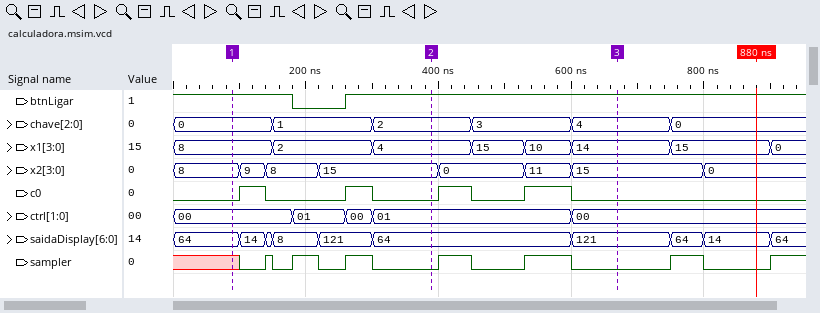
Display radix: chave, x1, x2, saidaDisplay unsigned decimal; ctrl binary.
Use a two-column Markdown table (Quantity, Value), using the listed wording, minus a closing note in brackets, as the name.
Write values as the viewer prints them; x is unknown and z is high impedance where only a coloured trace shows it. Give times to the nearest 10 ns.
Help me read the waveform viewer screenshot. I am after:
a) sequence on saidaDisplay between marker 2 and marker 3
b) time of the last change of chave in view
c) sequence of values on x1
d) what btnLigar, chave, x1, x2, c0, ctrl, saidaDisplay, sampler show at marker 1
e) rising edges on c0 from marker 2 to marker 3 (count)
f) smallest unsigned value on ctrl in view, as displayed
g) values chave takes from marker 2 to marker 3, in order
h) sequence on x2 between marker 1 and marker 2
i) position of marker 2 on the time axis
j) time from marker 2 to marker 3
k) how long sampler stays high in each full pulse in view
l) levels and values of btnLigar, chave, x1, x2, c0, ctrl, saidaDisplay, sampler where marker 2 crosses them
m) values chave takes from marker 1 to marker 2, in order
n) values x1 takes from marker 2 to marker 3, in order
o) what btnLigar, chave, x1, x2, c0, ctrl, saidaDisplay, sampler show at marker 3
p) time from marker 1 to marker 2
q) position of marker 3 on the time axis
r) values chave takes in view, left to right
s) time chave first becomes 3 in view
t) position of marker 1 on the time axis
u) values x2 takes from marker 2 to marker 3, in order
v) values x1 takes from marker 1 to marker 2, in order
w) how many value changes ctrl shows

| Quantity | Value |
|---|---|
| sequence on saidaDisplay between marker 2 and marker 3 | 64, 121 |
| time of the last change of chave in view | 750 ns |
| sequence of values on x1 | 8, 2, 4, 15, 10, 14, 15, 0 |
| what btnLigar, chave, x1, x2, c0, ctrl, saidaDisplay, sampler show at marker 1 | btnLigar=1, chave=0, x1=8, x2=8, c0=0, ctrl=00, saidaDisplay=64, sampler=x |
| rising edges on c0 from marker 2 to marker 3 | 2 |
| smallest unsigned value on ctrl in view, as displayed | 00 |
| values chave takes from marker 2 to marker 3, in order | 2, 3, 4 |
| sequence on x2 between marker 1 and marker 2 | 8, 9, 8, 15 |
| position of marker 2 on the time axis | 390 ns |
| time from marker 2 to marker 3 | 280 ns |
| how long sampler stays high in each full pulse in view | 10 ns, 40 ns, 40 ns, 50 ns, 70 ns, 50 ns |
| levels and values of btnLigar, chave, x1, x2, c0, ctrl, saidaDisplay, sampler where marker 2 crosses them | btnLigar=1, chave=2, x1=4, x2=15, c0=0, ctrl=01, saidaDisplay=64, sampler=0 |
| values chave takes from marker 1 to marker 2, in order | 0, 1, 2 |
| values x1 takes from marker 2 to marker 3, in order | 4, 15, 10, 14 |
| what btnLigar, chave, x1, x2, c0, ctrl, saidaDisplay, sampler show at marker 3 | btnLigar=1, chave=4, x1=14, x2=15, c0=0, ctrl=00, saidaDisplay=121, sampler=0 |
| time from marker 1 to marker 2 | 300 ns |
| position of marker 3 on the time axis | 670 ns |
| values chave takes in view, left to right | 0, 1, 2, 3, 4, 0 |
| time chave first becomes 3 in view | 450 ns |
| position of marker 1 on the time axis | 90 ns |
| values x2 takes from marker 2 to marker 3, in order | 15, 0, 11, 15 |
| values x1 takes from marker 1 to marker 2, in order | 8, 2, 4 |
| how many value changes ctrl shows | 4 |
